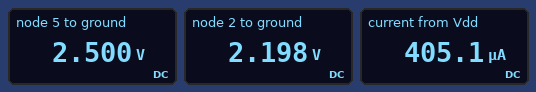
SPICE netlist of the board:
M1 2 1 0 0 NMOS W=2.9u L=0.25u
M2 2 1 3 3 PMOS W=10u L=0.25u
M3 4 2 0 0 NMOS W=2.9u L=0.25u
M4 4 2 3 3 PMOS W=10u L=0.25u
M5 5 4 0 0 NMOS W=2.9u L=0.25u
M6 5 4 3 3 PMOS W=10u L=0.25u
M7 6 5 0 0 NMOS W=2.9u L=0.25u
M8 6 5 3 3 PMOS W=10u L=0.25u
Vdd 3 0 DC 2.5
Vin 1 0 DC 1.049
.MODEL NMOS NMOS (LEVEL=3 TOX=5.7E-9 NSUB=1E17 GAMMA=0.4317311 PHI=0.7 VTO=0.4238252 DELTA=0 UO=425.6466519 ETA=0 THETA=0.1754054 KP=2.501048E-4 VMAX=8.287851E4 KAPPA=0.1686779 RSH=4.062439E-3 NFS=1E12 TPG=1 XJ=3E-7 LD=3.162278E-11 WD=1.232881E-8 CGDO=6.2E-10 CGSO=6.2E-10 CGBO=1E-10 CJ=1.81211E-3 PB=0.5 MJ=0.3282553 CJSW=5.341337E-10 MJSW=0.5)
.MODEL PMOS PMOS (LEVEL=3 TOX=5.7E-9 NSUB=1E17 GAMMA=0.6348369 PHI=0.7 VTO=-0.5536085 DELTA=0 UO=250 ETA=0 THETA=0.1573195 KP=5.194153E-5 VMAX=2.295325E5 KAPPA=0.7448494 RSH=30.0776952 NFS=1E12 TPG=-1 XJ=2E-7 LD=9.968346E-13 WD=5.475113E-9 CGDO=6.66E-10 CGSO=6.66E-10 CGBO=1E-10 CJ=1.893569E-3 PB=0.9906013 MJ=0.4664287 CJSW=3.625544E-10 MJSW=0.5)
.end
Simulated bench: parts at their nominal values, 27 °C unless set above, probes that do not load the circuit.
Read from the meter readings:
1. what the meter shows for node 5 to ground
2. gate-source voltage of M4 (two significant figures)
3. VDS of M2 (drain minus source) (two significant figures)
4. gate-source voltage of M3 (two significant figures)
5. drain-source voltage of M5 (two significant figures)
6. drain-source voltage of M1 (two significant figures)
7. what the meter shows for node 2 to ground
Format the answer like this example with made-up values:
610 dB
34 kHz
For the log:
2.500 V
-300 mV
-300 mV
2.2 V
2.5 V
2.2 V
2.198 V
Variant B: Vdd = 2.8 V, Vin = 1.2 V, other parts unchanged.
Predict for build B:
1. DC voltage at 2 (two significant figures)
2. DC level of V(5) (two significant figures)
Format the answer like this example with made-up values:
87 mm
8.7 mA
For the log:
2.4 V
2.8 V
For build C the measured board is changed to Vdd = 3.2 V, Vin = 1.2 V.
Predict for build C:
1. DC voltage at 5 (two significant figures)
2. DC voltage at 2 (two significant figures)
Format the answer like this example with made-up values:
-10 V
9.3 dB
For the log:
3.2 V
2.9 V
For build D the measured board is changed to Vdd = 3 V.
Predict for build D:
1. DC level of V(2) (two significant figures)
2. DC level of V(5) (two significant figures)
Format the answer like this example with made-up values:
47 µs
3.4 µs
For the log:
2.8 V
3.0 V
